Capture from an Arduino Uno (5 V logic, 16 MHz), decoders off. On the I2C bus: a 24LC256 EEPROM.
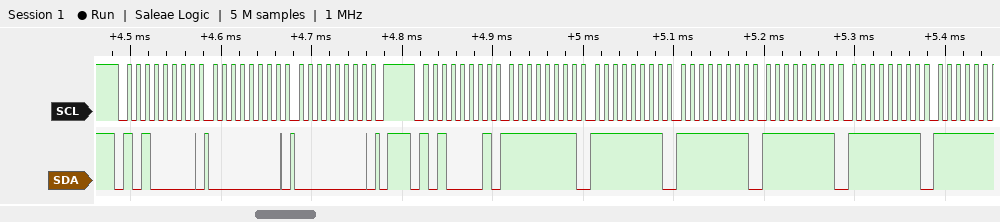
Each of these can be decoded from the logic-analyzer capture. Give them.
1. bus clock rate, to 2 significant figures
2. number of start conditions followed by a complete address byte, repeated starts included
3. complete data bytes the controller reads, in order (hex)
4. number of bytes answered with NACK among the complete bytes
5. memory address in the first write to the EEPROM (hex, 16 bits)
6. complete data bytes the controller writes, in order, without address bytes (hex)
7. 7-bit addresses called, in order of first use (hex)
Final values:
100 kHz
2
FF FF FF FF FF
0
0x0000
00 00
0x50
